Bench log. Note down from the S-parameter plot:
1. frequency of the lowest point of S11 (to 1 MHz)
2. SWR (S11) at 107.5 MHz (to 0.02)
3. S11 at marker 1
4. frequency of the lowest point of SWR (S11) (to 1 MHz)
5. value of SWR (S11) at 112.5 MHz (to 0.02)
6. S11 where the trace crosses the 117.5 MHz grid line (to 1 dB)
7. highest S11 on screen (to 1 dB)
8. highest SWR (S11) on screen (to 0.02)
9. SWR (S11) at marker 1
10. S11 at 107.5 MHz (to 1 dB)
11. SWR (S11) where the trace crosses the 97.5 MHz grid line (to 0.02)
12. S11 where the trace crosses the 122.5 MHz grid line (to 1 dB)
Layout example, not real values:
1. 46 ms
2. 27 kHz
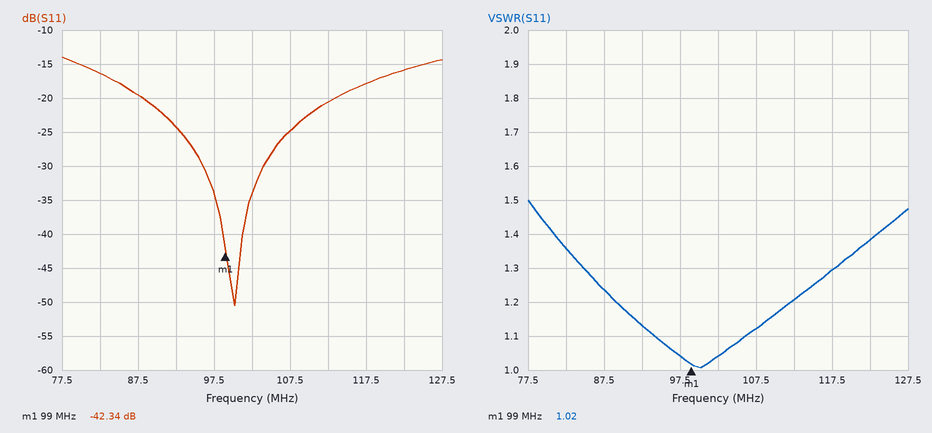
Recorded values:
1. 100 MHz
2. 1.12
3. -42.34 dB
4. 100 MHz
5. 1.20
6. -18 dB
7. -14 dB
8. 1.50
9. 1.02
10. -25 dB
11. 1.04
12. -16 dB
